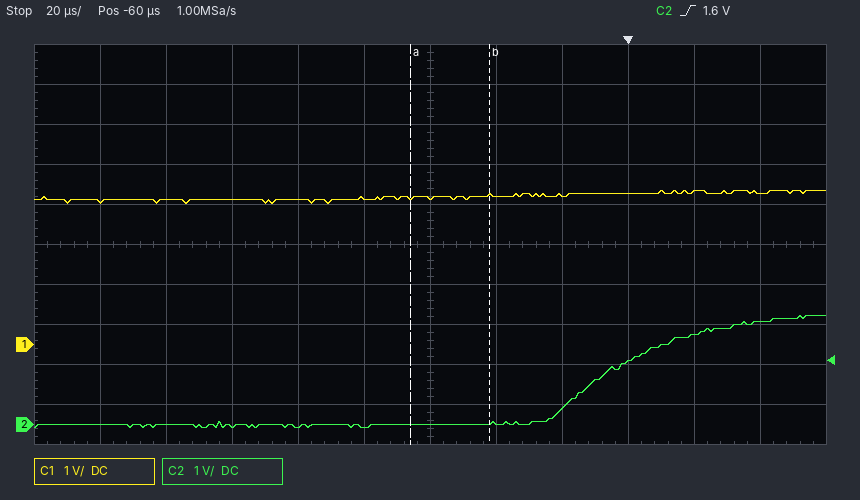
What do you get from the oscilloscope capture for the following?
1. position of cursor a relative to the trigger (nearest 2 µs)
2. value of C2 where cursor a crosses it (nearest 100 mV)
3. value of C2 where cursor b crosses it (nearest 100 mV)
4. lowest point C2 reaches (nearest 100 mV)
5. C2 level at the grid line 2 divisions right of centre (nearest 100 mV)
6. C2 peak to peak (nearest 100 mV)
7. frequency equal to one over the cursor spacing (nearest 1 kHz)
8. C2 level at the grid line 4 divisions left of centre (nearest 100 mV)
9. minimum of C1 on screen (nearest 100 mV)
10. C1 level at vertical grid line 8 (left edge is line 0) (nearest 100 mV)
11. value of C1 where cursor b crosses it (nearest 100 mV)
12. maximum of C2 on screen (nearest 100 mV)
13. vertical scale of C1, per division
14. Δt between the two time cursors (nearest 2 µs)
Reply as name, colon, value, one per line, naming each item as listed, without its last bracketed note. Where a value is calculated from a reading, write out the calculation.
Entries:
position of cursor a relative to the trigger: -66 µs
value of C2 where cursor a crosses it: 0.0 V
value of C2 where cursor b crosses it: 0.0 V
lowest point C2 reaches: -100 mV
C2 level at the grid line 2 divisions right of centre: 400 mV
C2 peak to peak: 2.7 V − (-100 mV) = 2.8 V
frequency equal to one over the cursor spacing: 1 / 24 µs ≈ 42 kHz
C2 level at the grid line 4 divisions left of centre: 0.0 V
minimum of C1 on screen: 3.5 V
C1 level at vertical grid line 8 (left edge is line 0): 3.7 V
value of C1 where cursor b crosses it: 3.7 V
maximum of C2 on screen: 2.7 V
vertical scale of C1, per division: 1 V
Δt between the two time cursors: 24 µs
